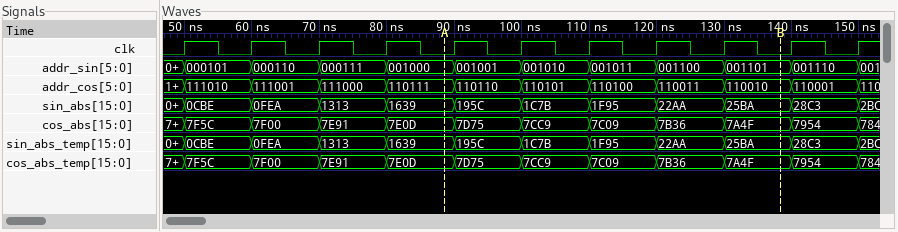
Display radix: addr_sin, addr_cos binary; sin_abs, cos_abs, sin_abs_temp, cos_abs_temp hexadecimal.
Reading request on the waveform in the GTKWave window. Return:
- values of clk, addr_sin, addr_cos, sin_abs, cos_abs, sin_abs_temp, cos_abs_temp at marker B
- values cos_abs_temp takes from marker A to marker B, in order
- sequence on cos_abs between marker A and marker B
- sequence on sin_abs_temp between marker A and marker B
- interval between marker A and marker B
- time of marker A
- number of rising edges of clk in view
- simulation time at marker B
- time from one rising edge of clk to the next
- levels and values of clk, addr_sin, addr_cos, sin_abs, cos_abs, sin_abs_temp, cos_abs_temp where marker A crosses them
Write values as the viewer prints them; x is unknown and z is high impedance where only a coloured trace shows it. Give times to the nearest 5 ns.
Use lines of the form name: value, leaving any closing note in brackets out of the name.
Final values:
values of clk, addr_sin, addr_cos, sin_abs, cos_abs, sin_abs_temp, cos_abs_temp at marker B: clk=0, addr_sin=001101, addr_cos=110010, sin_abs=25BA, cos_abs=7A4F, sin_abs_temp=25BA, cos_abs_temp=7A4F
values cos_abs_temp takes from marker A to marker B, in order: 7E0D, 7D75, 7CC9, 7C09, 7B36, 7A4F
sequence on cos_abs between marker A and marker B: 7E0D, 7D75, 7CC9, 7C09, 7B36, 7A4F
sequence on sin_abs_temp between marker A and marker B: 1639, 195C, 1C7B, 1F95, 22AA, 25BA
interval between marker A and marker B: 50 ns
time of marker A: 90 ns
number of rising edges of clk in view: 11
simulation time at marker B: 140 ns
time from one rising edge of clk to the next: 10 ns
levels and values of clk, addr_sin, addr_cos, sin_abs, cos_abs, sin_abs_temp, cos_abs_temp where marker A crosses them: clk=0, addr_sin=001000, addr_cos=110111, sin_abs=1639, cos_abs=7E0D, sin_abs_temp=1639, cos_abs_temp=7E0D
